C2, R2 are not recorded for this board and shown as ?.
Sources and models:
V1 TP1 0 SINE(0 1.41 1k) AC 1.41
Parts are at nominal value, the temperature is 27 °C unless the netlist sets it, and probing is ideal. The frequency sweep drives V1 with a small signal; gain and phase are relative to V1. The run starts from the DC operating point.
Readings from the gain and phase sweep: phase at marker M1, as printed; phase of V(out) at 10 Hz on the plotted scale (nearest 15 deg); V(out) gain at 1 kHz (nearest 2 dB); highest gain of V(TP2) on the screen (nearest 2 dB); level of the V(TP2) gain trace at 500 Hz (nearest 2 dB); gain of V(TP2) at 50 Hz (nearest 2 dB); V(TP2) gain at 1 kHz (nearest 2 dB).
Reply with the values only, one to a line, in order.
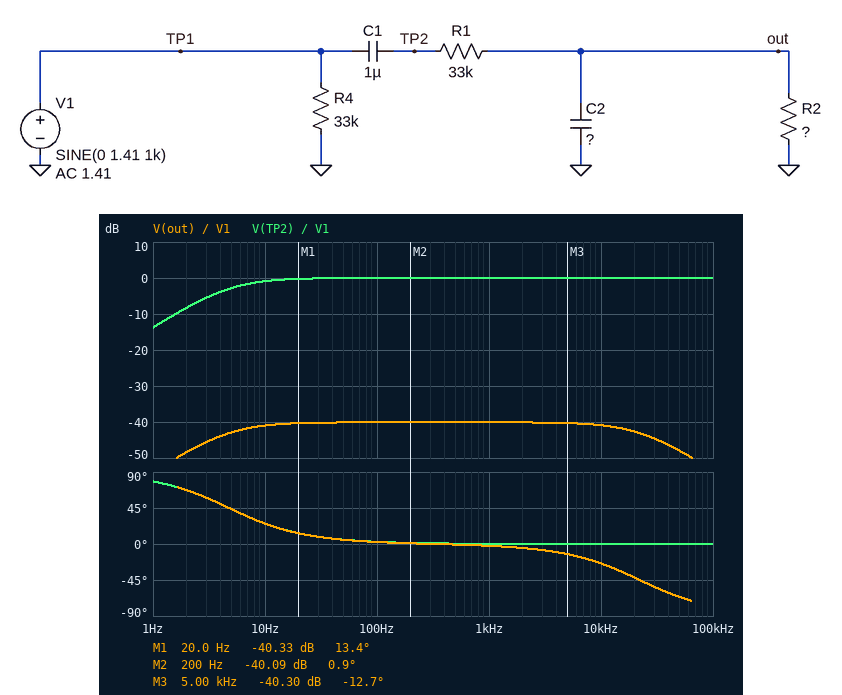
13.4 deg
30 deg
-40 dB
0 dB
0 dB
0 dB
0 dB
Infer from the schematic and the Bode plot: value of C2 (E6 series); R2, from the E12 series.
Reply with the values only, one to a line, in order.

22 nF
330 Ω
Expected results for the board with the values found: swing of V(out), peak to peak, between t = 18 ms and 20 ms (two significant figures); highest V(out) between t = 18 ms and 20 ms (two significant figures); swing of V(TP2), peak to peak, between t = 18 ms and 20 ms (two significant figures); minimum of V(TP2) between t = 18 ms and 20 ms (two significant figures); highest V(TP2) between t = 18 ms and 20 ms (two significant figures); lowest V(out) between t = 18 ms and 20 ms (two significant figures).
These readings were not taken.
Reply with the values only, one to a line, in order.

28 mV
14 mV
2.8 V
-1.4 V
1.4 V
-14 mV
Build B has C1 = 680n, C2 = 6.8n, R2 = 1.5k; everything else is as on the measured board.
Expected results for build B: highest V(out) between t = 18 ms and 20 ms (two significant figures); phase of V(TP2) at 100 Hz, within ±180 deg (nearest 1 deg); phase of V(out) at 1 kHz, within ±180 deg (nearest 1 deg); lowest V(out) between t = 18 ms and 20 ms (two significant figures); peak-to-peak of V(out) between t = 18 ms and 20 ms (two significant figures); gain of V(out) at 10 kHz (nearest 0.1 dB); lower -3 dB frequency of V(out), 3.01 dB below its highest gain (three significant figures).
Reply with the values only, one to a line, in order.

61 mV
4 deg
-3 deg
-61 mV
120 mV
-28.6 dB
6.78 Hz
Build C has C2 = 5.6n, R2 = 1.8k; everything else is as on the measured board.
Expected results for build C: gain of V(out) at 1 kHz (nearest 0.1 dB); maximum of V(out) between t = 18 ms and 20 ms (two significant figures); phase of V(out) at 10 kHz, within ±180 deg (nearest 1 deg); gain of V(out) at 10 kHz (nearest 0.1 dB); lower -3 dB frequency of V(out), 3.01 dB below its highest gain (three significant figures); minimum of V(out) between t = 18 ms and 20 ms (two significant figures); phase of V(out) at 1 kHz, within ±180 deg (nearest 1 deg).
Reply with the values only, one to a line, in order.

-25.7 dB
73 mV
-31 deg
-27.1 dB
4.57 Hz
-73 mV
-3 deg
